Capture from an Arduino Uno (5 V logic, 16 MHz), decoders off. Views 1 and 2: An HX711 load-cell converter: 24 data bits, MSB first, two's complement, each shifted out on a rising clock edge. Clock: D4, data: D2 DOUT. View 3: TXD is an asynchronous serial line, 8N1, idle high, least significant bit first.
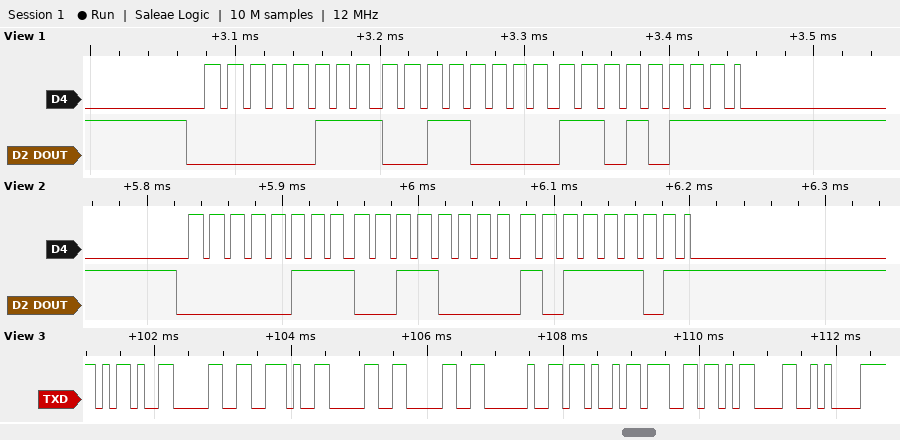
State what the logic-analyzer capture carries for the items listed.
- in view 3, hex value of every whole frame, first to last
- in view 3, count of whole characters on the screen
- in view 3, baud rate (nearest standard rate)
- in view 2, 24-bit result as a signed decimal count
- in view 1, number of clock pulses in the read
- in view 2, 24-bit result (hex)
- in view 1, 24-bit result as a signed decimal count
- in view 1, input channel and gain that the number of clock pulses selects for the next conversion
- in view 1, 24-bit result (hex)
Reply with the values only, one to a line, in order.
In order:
2D 30 2E 30 30 20 4B 67 0D 0A
10
9600 baud
471229
25
0x0730BD
471255
channel A, gain 128
0x0730D7
